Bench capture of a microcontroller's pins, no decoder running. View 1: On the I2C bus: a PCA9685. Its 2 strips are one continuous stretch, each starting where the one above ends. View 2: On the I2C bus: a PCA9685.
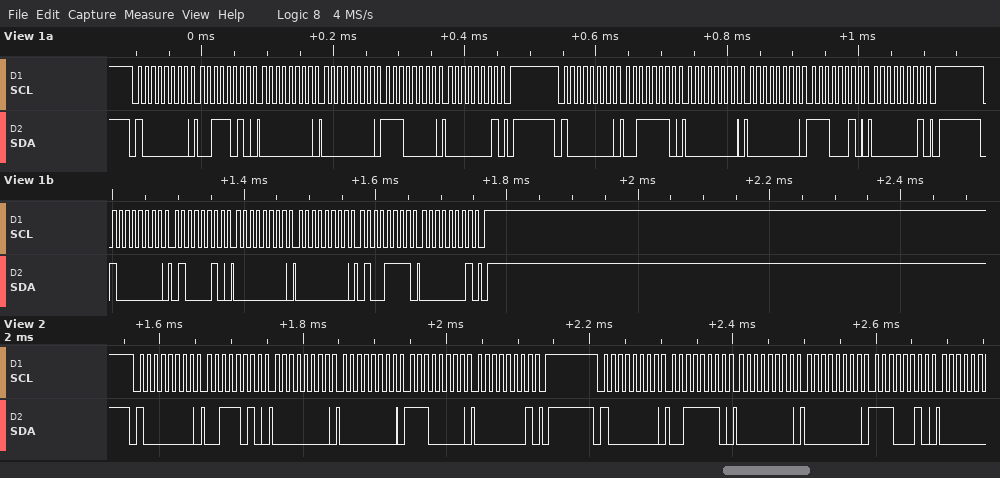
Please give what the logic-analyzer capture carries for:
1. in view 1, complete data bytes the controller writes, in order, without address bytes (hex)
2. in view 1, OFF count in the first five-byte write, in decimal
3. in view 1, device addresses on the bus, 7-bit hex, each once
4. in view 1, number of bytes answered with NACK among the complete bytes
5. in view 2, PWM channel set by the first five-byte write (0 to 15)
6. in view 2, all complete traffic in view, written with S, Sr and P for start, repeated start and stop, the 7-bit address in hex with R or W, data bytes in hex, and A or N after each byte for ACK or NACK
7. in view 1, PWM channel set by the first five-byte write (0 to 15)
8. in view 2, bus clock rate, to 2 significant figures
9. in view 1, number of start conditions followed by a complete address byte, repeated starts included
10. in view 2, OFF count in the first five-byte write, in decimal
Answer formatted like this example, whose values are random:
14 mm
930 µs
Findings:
3A 00 00 E0 01 3E 00 00 E2 01 42 00 00 4F 01
480
0x40
0
13
S 40W A 3A A 00 A 00 A E0 A 01 A P S 40W A 3E A 00 A 00 A E2 A
13
100 kHz
3
480
